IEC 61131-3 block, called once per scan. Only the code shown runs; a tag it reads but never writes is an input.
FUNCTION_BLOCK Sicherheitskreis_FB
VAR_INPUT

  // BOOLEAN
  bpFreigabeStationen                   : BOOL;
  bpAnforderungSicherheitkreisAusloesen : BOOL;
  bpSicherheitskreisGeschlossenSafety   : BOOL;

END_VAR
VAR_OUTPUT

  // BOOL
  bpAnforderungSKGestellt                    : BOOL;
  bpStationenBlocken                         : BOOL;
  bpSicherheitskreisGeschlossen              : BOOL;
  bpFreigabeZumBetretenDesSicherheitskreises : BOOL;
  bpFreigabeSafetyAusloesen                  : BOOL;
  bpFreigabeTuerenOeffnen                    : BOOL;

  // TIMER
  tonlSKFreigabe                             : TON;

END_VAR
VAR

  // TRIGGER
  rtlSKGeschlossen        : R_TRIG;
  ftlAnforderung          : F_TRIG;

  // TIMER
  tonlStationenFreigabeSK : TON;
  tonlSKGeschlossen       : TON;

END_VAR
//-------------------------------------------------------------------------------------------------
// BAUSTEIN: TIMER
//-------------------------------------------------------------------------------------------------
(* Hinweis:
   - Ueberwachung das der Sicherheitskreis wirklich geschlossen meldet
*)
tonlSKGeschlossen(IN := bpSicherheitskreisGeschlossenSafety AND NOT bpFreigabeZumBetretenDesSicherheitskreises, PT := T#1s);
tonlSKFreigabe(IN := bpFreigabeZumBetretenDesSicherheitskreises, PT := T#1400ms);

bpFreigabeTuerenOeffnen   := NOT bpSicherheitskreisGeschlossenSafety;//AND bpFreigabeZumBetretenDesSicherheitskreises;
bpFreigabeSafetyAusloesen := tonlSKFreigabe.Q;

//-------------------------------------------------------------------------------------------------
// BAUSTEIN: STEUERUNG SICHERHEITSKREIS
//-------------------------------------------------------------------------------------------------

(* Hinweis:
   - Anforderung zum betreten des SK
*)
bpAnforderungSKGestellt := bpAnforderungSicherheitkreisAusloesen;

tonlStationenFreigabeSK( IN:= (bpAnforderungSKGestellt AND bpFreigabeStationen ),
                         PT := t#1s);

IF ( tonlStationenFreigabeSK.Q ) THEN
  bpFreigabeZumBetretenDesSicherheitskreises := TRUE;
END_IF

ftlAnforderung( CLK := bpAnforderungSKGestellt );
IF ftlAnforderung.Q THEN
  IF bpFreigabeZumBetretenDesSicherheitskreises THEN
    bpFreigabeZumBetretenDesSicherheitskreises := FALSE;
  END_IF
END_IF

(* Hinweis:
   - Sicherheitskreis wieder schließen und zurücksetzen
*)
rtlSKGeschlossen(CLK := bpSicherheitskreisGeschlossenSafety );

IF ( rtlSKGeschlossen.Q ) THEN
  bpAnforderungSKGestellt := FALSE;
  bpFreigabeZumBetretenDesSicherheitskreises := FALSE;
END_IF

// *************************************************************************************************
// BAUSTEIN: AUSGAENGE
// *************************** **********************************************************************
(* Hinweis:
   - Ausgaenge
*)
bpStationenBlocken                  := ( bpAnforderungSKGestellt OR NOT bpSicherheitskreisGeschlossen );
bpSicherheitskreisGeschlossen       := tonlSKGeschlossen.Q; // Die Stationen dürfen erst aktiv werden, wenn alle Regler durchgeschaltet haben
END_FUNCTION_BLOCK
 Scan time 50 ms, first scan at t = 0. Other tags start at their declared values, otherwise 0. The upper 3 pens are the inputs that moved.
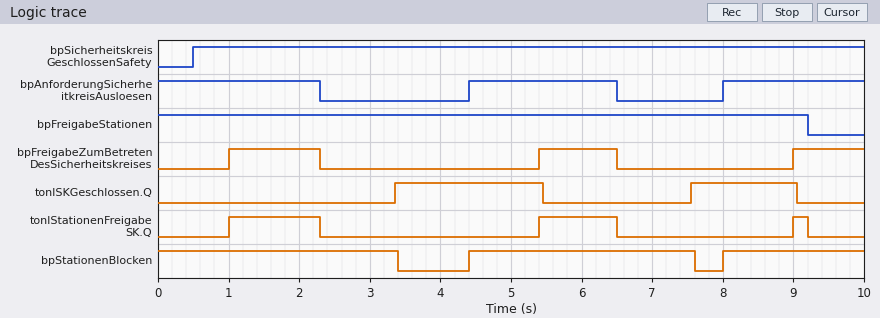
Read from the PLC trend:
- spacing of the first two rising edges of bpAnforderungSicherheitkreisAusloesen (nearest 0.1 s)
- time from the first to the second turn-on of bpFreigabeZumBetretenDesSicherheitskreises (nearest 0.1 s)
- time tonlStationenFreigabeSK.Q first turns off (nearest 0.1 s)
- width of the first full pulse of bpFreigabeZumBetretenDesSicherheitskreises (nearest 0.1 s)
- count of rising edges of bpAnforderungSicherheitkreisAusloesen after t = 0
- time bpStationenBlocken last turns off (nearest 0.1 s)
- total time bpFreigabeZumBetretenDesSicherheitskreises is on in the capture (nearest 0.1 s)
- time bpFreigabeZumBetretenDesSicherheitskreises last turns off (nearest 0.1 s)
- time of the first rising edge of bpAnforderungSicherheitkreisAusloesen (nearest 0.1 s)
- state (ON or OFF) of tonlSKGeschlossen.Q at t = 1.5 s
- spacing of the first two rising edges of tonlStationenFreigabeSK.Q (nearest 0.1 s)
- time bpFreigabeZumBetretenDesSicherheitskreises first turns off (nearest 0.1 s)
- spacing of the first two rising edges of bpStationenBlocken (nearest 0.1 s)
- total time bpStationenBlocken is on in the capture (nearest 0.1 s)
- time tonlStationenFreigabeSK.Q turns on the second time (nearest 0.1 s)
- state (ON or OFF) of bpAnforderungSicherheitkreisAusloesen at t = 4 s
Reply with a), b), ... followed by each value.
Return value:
a) 3.6 s
b) 4.4 s
c) 2.3 s
d) 1.3 s
e) 2
f) 7.6 s
g) 3.4 s
h) 6.5 s
i) 4.4 s
j) OFF
k) 4.4 s
l) 2.3 s
m) 3.6 s
n) 8.6 s
o) 5.4 s
p) OFF
